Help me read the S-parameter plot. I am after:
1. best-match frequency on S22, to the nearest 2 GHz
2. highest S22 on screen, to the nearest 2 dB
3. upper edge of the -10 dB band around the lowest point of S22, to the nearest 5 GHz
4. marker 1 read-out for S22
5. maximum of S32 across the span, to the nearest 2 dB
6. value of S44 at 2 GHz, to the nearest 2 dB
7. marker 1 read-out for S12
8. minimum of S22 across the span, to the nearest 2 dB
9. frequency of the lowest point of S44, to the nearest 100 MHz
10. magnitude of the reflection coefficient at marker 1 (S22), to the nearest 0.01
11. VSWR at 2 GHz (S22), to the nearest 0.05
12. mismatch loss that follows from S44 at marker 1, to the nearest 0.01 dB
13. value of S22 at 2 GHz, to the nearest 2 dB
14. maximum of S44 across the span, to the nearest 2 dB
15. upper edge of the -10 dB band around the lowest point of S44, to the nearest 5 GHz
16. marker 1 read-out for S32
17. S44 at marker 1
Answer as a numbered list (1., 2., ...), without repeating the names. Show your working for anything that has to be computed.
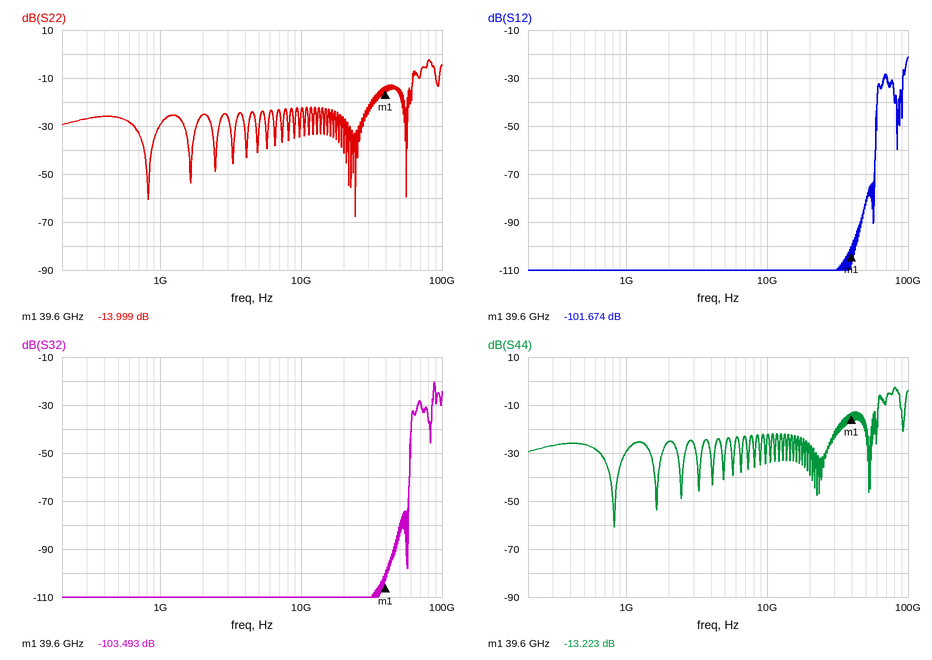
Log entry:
1. 24 GHz
2. -2 dB
3. 60 GHz
4. -13.999 dB
5. -20 dB
6. -26 dB
7. -101.674 dB
8. -68 dB
9. 800 MHz
10. 10^(-13.999/20) ≈ 0.20
11. |Γ| = 10^(-26/20) = 0.0501; VSWR = (1 + 0.0501)/(1 − 0.0501) ≈ 1.11, so 1.10 to the nearest 0.05
12. −10 log10(1 − 10^(-13.223/10)) ≈ 0.21 dB
13. -26 dB
14. -2 dB
15. 60 GHz
16. -103.493 dB
17. -13.223 dB
